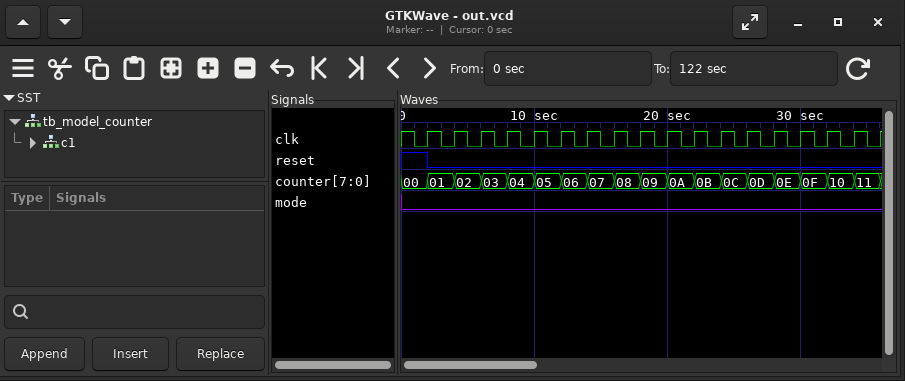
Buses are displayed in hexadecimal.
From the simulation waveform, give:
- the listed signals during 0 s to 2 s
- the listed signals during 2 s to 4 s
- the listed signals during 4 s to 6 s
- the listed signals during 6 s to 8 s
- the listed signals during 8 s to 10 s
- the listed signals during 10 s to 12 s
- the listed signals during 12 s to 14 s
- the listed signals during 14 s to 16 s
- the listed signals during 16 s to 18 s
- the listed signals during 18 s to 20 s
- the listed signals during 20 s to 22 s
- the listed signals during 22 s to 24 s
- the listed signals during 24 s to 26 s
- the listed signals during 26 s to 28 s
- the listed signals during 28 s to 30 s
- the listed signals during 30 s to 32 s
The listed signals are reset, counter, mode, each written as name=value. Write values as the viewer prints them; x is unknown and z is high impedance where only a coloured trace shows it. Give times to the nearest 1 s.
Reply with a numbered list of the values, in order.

1. reset=1, counter=00, mode=0
2. reset=0, counter=01, mode=0
3. reset=0, counter=02, mode=0
4. reset=0, counter=03, mode=0
5. reset=0, counter=04, mode=0
6. reset=0, counter=05, mode=0
7. reset=0, counter=06, mode=0
8. reset=0, counter=07, mode=0
9. reset=0, counter=08, mode=0
10. reset=0, counter=09, mode=0
11. reset=0, counter=0A, mode=0
12. reset=0, counter=0B, mode=0
13. reset=0, counter=0C, mode=0
14. reset=0, counter=0D, mode=0
15. reset=0, counter=0E, mode=0
16. reset=0, counter=0F, mode=0
